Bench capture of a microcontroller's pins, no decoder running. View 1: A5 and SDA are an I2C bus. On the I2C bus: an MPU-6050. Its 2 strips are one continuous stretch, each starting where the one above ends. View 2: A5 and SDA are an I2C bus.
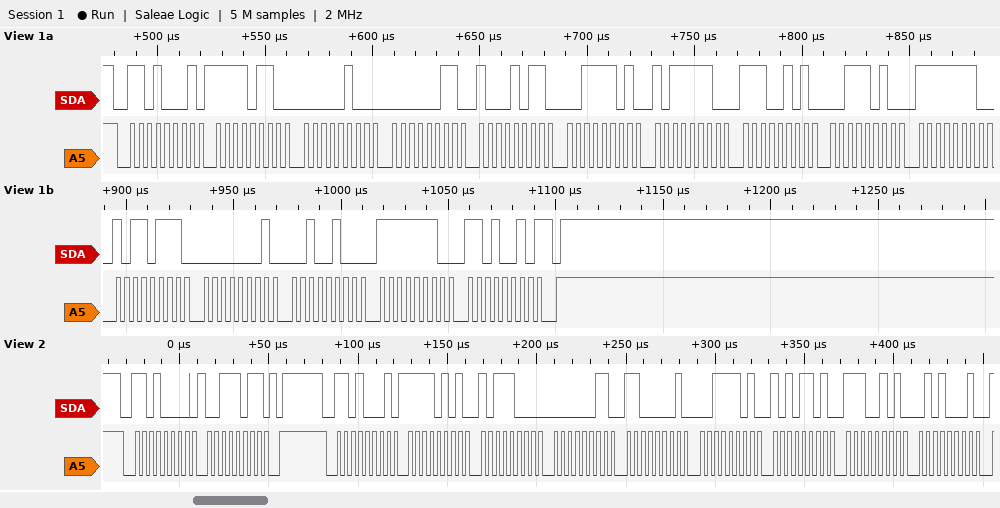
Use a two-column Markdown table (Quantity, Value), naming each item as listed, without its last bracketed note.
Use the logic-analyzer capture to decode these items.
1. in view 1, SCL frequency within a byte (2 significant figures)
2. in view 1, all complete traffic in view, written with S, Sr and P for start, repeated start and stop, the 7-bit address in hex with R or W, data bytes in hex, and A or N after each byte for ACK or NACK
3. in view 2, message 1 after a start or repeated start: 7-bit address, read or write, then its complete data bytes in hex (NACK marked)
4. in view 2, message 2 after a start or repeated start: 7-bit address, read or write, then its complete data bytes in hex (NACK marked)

| Quantity | Value |
|---|---|
| in view 1, SCL frequency within a byte | 250 kHz |
| in view 1, all complete traffic in view, written with S, Sr and P for start, repeated start and stop, the 7-bit address in hex with R or W, data bytes in hex, and A or N after each byte for ACK or NACK | S 68R A F6 A 04 A 03 A 8B A 3D A BE A E5 A 3A A FE A B7 A 01 A 24 A FE A D2 N P |
| in view 2, message 1 after a start or repeated start: 7-bit address, read or write, then its complete data bytes in hex | 0x68 write: 3B |
| in view 2, message 2 after a start or repeated start: 7-bit address, read or write, then its complete data bytes in hex | 0x68 read: F5 B8 03 C1 3D AD E5 51 |
